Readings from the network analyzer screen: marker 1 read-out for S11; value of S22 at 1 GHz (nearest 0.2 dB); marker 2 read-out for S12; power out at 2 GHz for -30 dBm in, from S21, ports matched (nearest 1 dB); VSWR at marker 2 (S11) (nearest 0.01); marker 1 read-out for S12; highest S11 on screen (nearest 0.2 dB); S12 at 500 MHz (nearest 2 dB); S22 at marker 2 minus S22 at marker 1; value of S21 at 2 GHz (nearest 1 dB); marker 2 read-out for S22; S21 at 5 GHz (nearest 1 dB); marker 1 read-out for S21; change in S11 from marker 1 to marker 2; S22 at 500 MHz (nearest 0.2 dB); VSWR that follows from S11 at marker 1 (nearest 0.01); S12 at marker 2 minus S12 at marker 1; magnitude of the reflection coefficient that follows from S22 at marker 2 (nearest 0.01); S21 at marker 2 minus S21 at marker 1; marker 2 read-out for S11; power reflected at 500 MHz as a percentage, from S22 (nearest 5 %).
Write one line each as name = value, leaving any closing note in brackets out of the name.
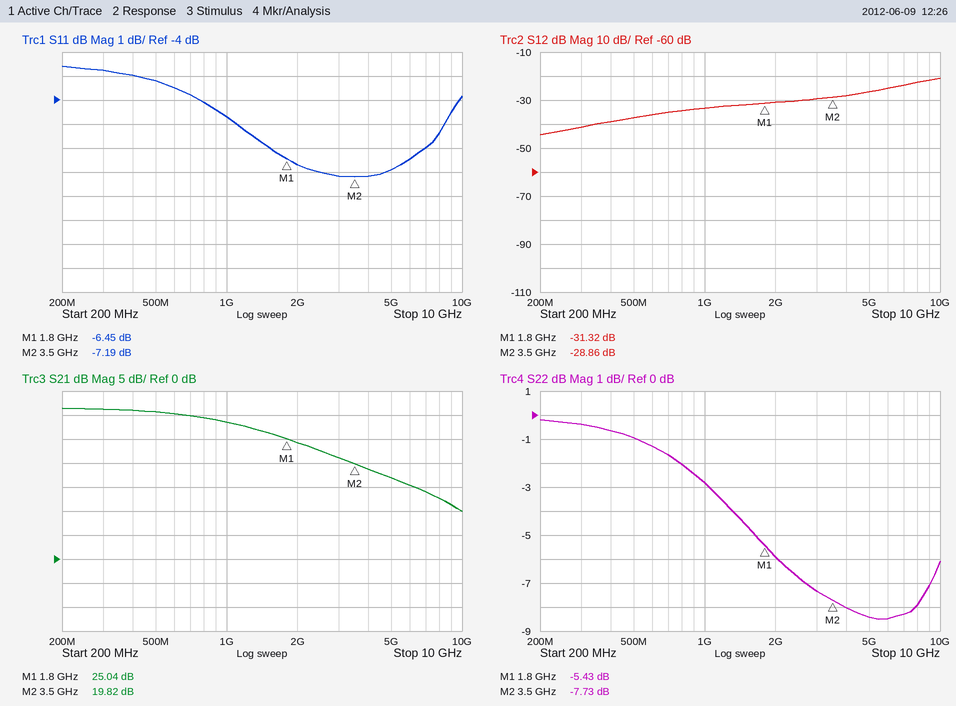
marker 1 read-out for S11 = -6.45 dB
value of S22 at 1 GHz = -2.8 dB
marker 2 read-out for S12 = -28.86 dB
power out at 2 GHz for -30 dBm in, from S21, ports matched = -6 dBm
VSWR at marker 2 (S11) = 2.55
marker 1 read-out for S12 = -31.32 dB
highest S11 on screen = -2.6 dB
S12 at 500 MHz = -38 dB
S22 at marker 2 minus S22 at marker 1 = -2.30 dB
value of S21 at 2 GHz = 24 dB
marker 2 read-out for S22 = -7.73 dB
S21 at 5 GHz = 17 dB
marker 1 read-out for S21 = 25.04 dB
change in S11 from marker 1 to marker 2 = -0.74 dB
S22 at 500 MHz = -1.0 dB
VSWR that follows from S11 at marker 1 = 2.82
S12 at marker 2 minus S12 at marker 1 = 2.46 dB
magnitude of the reflection coefficient that follows from S22 at marker 2 = 0.41
S21 at marker 2 minus S21 at marker 1 = -5.22 dB
marker 2 read-out for S11 = -7.19 dB
power reflected at 500 MHz as a percentage, from S22 = 80 %
